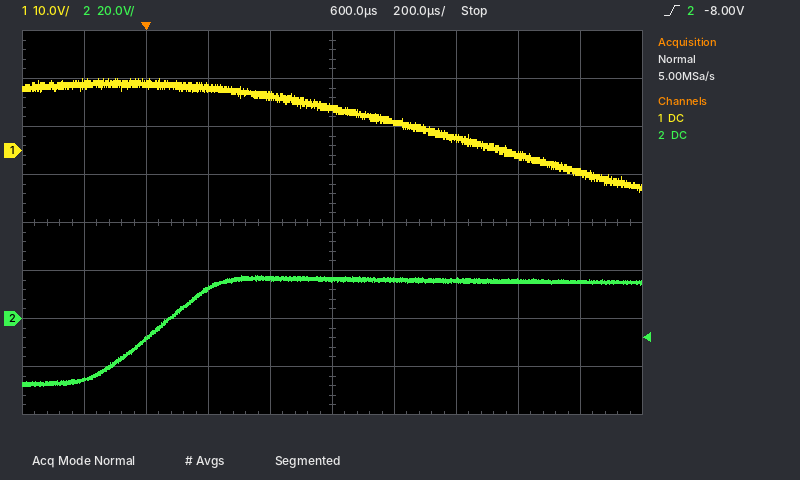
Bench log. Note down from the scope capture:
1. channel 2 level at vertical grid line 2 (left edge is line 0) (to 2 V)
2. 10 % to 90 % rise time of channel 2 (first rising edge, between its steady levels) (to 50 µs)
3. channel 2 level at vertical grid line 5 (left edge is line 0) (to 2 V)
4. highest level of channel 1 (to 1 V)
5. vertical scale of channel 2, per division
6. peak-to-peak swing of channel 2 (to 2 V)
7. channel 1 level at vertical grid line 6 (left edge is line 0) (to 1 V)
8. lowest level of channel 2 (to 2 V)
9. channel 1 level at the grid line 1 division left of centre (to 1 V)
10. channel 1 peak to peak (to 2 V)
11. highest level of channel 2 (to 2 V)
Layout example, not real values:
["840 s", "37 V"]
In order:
["-8 V", "350 µs", "16 V", "15 V", "20 V", "46 V", "6 V", "-28 V", "11 V", "24 V", "18 V"]
